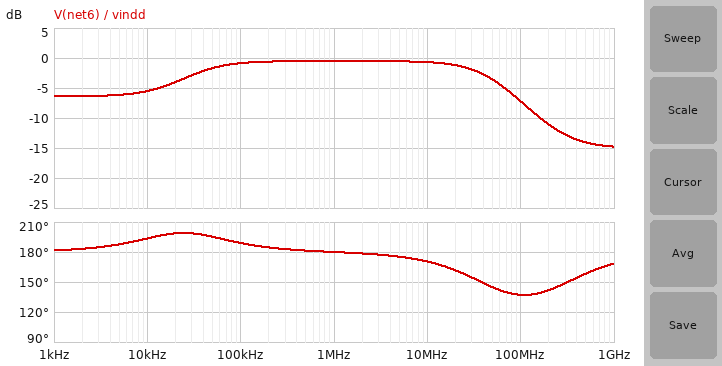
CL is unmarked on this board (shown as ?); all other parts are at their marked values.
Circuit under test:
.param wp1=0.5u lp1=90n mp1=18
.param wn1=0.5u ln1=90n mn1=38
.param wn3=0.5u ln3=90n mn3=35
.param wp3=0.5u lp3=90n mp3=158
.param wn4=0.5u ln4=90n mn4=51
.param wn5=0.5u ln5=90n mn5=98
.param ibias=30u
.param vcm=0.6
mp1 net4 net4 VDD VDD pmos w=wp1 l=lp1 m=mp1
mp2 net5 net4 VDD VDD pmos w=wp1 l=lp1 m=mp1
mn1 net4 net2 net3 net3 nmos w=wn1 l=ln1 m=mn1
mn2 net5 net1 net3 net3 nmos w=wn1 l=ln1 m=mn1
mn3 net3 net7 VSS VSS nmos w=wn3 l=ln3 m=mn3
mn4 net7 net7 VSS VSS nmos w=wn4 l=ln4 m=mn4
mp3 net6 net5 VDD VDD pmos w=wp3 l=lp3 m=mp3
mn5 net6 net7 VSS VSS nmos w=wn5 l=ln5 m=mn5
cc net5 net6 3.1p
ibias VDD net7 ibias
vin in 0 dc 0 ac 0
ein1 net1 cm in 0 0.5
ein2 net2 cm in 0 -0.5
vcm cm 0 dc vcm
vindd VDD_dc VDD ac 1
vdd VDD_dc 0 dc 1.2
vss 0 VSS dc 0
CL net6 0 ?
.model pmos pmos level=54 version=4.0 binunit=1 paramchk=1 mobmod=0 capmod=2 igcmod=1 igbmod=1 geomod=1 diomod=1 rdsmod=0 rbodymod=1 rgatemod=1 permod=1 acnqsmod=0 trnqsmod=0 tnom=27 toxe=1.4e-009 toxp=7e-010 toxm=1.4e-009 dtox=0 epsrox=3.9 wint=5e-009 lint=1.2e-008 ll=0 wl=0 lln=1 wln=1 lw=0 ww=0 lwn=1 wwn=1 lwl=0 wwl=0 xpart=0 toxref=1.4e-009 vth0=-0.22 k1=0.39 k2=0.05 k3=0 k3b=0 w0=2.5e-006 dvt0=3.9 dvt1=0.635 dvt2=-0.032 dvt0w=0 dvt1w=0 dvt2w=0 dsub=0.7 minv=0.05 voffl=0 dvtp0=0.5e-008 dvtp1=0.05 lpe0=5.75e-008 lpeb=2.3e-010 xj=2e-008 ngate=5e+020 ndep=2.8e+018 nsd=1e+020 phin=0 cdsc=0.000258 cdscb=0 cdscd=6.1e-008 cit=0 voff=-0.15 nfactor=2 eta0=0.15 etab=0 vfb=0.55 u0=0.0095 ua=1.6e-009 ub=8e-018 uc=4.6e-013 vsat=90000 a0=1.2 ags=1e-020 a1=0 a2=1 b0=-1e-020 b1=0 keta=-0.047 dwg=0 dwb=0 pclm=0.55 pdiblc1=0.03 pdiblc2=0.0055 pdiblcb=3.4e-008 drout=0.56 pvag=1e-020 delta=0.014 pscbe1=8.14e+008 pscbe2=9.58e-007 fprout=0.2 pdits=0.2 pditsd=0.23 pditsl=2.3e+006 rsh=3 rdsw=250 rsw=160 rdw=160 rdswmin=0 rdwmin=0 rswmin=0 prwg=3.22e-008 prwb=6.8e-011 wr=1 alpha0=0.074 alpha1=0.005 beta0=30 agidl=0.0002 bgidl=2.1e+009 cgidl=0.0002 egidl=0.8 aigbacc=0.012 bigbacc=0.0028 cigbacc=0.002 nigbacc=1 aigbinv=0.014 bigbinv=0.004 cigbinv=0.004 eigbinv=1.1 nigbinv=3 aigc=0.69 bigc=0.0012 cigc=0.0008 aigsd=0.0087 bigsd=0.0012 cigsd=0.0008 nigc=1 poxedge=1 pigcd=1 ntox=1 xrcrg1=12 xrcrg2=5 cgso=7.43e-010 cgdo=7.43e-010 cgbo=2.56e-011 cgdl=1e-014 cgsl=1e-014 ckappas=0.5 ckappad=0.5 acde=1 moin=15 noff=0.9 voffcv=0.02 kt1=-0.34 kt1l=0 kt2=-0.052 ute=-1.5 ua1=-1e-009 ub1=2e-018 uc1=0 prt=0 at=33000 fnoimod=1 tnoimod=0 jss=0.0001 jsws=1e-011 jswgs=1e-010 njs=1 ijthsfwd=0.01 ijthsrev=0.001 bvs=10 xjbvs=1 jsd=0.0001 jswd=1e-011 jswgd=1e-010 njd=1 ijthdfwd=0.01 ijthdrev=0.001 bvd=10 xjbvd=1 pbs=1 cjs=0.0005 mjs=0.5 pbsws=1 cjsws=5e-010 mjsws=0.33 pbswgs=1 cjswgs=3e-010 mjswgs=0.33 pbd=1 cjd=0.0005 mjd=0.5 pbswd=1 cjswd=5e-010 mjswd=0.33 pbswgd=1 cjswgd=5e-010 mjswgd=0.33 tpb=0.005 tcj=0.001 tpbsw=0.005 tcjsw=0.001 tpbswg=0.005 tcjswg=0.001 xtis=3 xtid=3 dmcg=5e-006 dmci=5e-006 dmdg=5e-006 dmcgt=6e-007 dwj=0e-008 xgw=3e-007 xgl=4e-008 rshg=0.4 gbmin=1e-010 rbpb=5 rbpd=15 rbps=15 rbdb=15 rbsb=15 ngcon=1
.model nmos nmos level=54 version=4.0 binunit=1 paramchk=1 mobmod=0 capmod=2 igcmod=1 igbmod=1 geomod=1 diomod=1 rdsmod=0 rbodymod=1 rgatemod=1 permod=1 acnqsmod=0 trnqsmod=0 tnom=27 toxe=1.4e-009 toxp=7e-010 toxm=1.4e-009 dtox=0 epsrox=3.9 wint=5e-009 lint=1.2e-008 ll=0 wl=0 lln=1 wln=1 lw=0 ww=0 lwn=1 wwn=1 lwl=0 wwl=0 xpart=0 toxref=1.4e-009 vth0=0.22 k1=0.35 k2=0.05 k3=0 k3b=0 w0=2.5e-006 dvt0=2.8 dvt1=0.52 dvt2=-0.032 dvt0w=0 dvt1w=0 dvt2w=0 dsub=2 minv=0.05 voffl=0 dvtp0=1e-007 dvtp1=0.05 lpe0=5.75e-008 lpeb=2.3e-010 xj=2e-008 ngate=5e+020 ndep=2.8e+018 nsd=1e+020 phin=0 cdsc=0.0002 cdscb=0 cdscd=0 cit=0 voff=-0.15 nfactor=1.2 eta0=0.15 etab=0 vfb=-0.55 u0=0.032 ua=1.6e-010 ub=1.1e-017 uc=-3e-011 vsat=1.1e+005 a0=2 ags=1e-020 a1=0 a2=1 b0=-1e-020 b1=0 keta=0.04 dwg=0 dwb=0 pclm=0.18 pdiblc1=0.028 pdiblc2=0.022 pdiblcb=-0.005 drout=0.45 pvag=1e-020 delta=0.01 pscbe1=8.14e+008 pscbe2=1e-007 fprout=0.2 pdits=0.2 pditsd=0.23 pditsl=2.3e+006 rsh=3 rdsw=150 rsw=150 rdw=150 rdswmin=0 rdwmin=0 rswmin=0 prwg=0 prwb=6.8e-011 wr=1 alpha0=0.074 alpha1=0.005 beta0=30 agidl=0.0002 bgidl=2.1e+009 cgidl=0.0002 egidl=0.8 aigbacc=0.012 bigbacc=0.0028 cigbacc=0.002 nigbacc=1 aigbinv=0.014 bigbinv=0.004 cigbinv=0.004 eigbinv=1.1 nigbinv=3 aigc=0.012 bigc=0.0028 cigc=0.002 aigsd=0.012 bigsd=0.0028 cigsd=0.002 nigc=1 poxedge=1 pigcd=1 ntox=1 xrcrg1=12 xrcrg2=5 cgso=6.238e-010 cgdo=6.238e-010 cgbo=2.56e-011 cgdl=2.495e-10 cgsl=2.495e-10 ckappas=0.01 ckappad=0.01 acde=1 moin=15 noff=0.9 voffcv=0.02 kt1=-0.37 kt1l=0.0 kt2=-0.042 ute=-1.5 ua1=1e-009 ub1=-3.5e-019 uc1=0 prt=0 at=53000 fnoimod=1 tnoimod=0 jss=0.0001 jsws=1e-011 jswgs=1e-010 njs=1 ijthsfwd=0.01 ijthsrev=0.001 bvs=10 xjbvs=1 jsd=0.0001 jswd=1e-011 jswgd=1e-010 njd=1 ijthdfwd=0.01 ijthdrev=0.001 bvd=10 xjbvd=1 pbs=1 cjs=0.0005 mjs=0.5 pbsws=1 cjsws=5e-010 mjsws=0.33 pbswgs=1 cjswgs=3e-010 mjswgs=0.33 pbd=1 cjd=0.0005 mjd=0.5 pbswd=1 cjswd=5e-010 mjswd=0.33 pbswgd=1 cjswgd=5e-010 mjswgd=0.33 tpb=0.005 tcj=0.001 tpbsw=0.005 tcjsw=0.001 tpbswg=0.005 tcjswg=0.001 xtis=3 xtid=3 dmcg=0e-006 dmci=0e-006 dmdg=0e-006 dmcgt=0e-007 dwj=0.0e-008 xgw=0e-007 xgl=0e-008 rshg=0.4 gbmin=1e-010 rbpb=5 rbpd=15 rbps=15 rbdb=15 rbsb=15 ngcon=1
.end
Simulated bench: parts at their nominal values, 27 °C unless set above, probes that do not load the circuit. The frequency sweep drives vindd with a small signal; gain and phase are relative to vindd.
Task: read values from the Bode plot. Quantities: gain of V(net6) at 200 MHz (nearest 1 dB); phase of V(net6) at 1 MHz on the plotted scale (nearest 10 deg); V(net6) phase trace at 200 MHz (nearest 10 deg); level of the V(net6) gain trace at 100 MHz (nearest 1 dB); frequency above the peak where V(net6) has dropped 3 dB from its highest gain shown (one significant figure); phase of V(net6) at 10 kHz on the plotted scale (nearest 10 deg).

-11 dB
180 deg
140 deg
-7 dB
50 MHz
190 deg
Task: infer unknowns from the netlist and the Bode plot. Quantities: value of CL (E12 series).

4.7 pF
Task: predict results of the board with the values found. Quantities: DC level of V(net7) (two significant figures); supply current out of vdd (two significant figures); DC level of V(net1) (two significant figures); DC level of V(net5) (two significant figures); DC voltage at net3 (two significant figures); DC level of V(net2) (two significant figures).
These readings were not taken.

300 mV
140 µA
600 mV
870 mV
340 mV
600 mV
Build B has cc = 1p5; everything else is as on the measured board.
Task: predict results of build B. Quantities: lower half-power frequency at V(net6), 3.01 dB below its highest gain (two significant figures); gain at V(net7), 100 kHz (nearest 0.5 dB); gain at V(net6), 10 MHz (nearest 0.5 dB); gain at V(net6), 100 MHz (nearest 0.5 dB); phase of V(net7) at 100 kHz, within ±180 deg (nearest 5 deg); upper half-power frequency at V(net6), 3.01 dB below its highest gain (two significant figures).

47 kHz
-39.0 dB
-1.0 dB
-7.5 dB
-165 deg
47 MHz
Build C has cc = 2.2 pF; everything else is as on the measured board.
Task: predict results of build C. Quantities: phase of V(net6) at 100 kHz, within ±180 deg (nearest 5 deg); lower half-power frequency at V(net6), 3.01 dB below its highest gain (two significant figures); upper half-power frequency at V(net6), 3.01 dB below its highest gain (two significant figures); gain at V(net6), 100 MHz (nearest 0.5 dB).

-170 deg
33 kHz
48 MHz
-7.5 dB
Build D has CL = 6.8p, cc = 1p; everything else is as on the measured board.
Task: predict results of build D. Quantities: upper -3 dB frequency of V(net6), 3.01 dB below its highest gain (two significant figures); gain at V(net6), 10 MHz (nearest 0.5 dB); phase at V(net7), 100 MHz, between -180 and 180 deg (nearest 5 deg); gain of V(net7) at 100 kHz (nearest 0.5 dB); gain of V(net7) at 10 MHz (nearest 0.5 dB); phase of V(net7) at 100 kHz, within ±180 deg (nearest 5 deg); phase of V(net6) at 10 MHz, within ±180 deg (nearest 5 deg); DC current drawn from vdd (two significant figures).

33 MHz
-1.0 dB
-170 deg
-39.5 dB
-38.0 dB
-165 deg
165 deg
140 µA
